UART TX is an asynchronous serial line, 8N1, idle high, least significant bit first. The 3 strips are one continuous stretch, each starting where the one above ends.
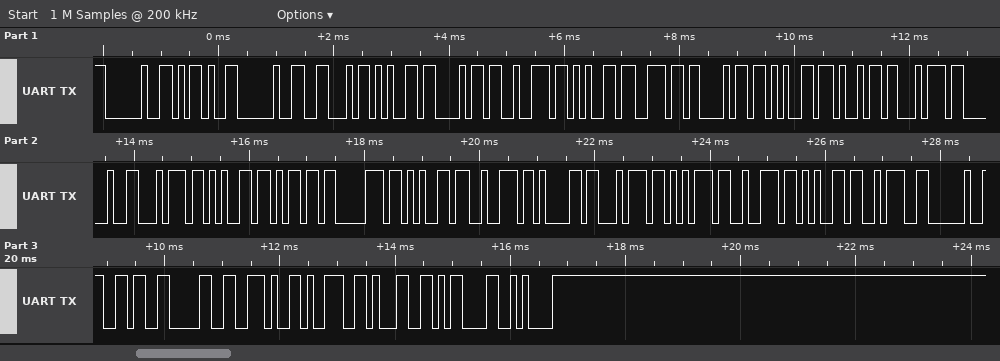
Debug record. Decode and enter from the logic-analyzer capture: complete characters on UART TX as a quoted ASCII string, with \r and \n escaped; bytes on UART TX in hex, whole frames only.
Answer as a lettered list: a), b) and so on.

a) " - Fehrenheit temperature: 60.91\r\n"
b) 20 2D 20 46 65 68 72 65 6E 68 65 69 74 20 74 65 6D 70 65 72 61 74 75 72 65 3A 20 36 30 2E 39 31 0D 0A
